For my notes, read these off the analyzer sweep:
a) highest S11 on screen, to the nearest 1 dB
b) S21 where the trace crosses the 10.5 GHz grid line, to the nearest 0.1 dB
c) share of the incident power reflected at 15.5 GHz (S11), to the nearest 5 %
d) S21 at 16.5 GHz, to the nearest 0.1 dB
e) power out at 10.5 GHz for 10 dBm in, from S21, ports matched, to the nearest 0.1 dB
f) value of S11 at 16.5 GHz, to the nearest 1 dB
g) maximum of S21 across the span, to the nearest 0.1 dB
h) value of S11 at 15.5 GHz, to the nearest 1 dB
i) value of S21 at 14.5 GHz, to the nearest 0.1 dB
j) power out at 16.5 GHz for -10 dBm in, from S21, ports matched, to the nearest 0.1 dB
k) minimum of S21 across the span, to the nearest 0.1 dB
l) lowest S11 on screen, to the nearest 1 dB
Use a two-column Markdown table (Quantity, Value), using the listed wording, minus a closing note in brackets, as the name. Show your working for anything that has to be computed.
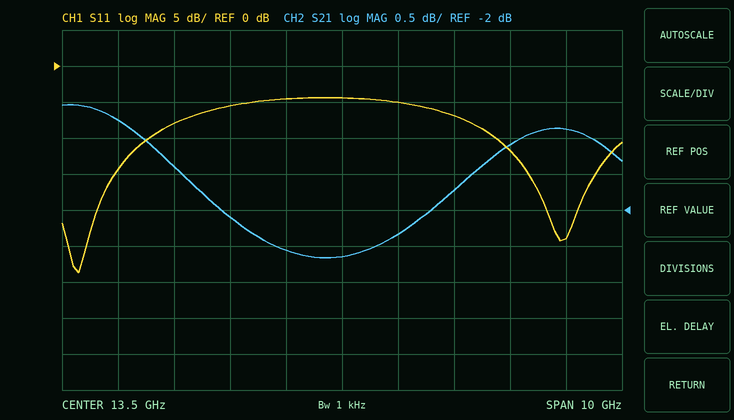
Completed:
| Quantity | Value |
|---|---|
| highest S11 on screen, to the nearest 1 dB | -4 dB |
| S21 where the trace crosses the 10.5 GHz grid line, to the nearest 0.1 dB | -1.4 dB |
| share of the incident power reflected at 15.5 GHz (S11), to the nearest 5 % | 10^(-7/10) ≈ 20 % |
| S21 at 16.5 GHz, to the nearest 0.1 dB | -1.1 dB |
| power out at 10.5 GHz for 10 dBm in, from S21, ports matched, to the nearest 0.1 dB | 10 dBm + (-1.4 dB) = 8.6 dBm |
| value of S11 at 16.5 GHz, to the nearest 1 dB | -12 dB |
| maximum of S21 across the span, to the nearest 0.1 dB | -0.5 dB |
| value of S11 at 15.5 GHz, to the nearest 1 dB | -7 dB |
| value of S21 at 14.5 GHz, to the nearest 0.1 dB | -2.3 dB |
| power out at 16.5 GHz for -10 dBm in, from S21, ports matched, to the nearest 0.1 dB | -10 dBm + (-1.1 dB) = -11.1 dBm |
| minimum of S21 across the span, to the nearest 0.1 dB | -2.7 dB |
| lowest S11 on screen, to the nearest 1 dB | -29 dB |
